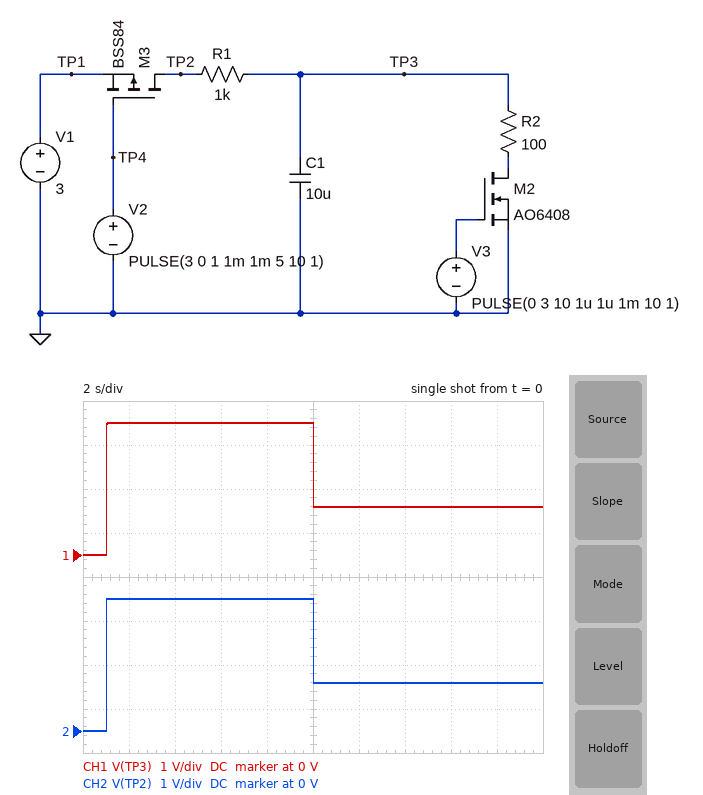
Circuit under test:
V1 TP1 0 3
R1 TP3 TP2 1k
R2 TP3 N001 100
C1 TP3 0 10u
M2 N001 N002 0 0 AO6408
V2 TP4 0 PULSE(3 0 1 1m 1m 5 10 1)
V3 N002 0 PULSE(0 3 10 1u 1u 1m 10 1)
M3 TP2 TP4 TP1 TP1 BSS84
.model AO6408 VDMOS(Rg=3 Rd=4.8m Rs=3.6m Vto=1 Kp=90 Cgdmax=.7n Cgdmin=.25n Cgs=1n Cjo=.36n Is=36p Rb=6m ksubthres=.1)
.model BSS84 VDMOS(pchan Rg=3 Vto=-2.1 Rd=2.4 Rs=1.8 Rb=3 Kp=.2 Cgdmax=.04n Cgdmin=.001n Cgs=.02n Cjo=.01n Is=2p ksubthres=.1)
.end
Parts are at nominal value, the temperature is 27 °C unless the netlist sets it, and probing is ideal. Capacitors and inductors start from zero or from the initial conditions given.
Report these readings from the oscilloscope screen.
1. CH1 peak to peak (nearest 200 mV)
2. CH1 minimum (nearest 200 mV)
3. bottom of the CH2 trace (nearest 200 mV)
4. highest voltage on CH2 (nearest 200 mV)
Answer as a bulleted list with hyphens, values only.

- 3.0 V
- 0 V
- 0 V
- 3.0 V
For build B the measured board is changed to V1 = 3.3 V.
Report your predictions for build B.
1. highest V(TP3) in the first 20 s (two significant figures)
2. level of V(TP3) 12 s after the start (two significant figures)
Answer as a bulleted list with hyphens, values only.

- 3.3 V
- 1.2 V
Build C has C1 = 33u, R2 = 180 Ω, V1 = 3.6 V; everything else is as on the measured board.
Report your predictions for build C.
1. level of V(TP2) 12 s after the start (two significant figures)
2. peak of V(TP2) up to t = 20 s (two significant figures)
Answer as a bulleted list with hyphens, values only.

- 3.0 V
- 3.6 V
